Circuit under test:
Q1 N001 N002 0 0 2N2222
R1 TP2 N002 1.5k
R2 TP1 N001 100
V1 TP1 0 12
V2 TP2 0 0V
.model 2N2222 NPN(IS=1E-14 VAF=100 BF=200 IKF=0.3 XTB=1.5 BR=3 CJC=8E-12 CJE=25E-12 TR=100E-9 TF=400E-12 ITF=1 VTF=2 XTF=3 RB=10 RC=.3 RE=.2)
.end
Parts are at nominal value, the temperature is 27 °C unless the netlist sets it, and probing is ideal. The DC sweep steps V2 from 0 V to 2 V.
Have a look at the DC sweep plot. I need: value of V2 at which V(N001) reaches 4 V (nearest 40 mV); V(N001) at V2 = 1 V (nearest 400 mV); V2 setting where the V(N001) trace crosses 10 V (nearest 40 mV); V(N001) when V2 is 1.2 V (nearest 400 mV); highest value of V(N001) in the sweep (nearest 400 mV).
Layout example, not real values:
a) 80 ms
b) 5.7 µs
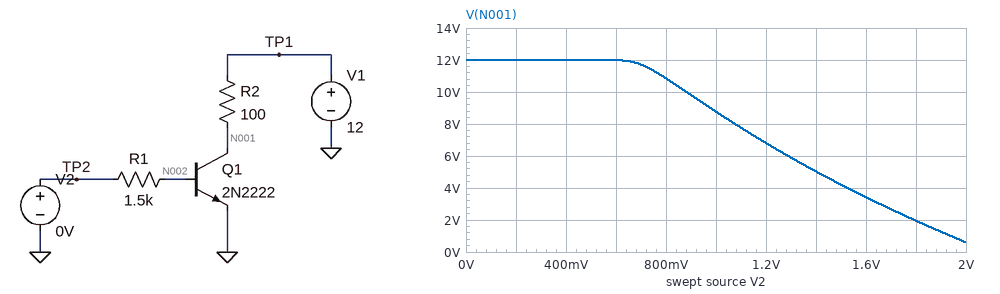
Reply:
a) 1.52 V
b) 8.8 V
c) 880 mV
d) 6.8 V
e) 12.0 V
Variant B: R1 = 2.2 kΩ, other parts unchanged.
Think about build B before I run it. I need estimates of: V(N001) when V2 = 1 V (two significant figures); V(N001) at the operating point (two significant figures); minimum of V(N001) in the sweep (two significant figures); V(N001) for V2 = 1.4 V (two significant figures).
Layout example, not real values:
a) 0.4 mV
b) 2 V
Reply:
a) 9.6 V
b) 12 V
c) 3.3 V
d) 6.8 V
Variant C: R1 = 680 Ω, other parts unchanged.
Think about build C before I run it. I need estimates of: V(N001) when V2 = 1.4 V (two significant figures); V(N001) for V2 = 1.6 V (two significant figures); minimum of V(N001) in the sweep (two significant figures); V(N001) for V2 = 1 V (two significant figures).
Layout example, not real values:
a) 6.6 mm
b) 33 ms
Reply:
a) 250 mV
b) 190 mV
c) 170 mV
d) 6.2 V
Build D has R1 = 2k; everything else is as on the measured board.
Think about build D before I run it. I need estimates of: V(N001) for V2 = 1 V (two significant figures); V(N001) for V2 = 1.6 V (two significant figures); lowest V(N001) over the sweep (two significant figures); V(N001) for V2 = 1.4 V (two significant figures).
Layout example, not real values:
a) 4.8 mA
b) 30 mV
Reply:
a) 9.4 V
b) 5.1 V
c) 2.7 V
d) 6.4 V
